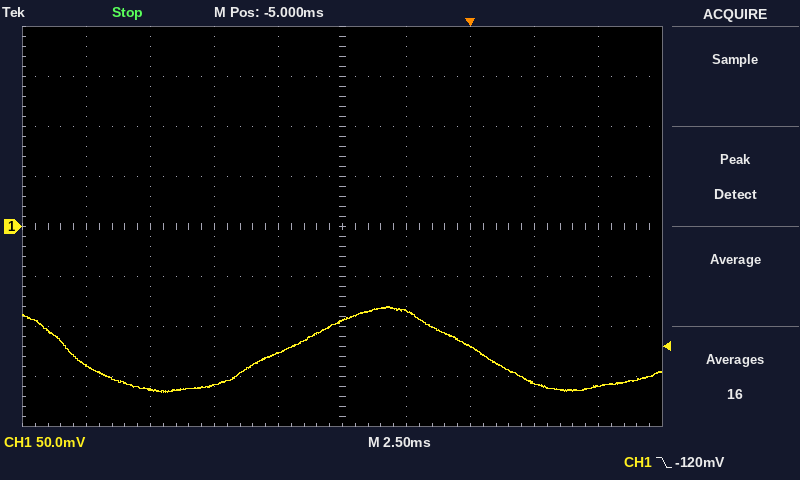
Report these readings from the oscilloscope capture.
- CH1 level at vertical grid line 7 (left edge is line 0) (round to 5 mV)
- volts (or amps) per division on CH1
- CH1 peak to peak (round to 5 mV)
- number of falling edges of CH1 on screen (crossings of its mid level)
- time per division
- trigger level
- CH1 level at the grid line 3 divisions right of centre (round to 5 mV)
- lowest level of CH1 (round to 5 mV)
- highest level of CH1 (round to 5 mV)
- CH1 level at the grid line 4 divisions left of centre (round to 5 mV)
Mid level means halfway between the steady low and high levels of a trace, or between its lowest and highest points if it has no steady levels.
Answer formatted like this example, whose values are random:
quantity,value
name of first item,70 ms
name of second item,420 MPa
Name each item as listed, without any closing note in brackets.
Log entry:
quantity,value
CH1 level at vertical grid line 7 (left edge is line 0),-120 mV
volts (or amps) per division on CH1,50 mV
CH1 peak to peak,85 mV
number of falling edges of CH1 on screen,2
time per division,2.5 ms
trigger level,-120 mV
CH1 level at the grid line 3 divisions right of centre,-155 mV
lowest level of CH1,-165 mV
highest level of CH1,-80 mV
CH1 level at the grid line 4 divisions left of centre,-140 mV
